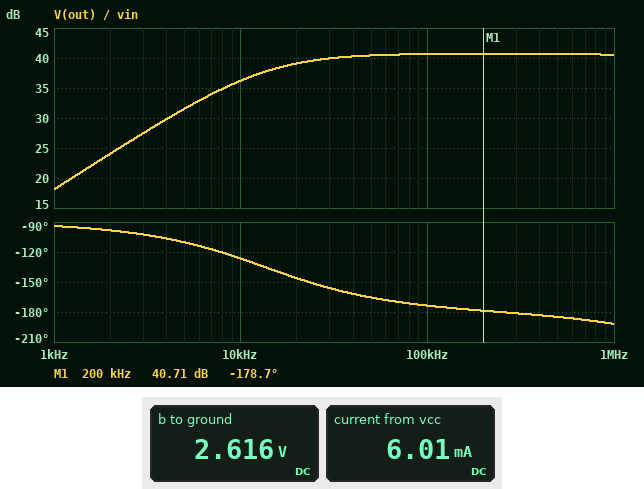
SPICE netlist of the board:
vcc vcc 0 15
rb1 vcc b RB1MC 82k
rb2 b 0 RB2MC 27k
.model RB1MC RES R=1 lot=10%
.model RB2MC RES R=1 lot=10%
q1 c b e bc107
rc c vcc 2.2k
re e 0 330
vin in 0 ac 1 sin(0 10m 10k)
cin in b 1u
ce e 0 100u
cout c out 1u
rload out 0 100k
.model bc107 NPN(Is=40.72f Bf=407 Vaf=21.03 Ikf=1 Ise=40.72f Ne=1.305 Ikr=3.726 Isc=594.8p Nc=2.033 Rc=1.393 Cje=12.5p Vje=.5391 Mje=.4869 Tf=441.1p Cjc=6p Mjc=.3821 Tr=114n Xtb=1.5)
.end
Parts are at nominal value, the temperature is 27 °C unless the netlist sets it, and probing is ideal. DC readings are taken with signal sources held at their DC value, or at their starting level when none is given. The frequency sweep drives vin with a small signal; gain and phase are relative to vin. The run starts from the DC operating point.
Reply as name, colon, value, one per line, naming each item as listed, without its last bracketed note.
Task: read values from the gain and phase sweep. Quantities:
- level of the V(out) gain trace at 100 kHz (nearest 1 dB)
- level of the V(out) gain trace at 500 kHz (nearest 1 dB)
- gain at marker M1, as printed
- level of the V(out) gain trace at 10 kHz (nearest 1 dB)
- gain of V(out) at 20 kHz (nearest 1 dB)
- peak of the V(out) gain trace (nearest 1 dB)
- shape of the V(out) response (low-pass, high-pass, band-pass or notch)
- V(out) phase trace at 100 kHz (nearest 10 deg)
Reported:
level of the V(out) gain trace at 100 kHz: 41 dB
level of the V(out) gain trace at 500 kHz: 41 dB
gain at marker M1, as printed: 40.71 dB
level of the V(out) gain trace at 10 kHz: 36 dB
gain of V(out) at 20 kHz: 39 dB
peak of the V(out) gain trace: 41 dB
shape of the V(out) response: high-pass
V(out) phase trace at 100 kHz: -170 deg
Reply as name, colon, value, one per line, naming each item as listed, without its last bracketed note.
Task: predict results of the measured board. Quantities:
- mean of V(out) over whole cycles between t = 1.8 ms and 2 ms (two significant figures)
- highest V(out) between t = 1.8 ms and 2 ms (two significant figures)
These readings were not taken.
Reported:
mean of V(out) over whole cycles between t = 1.8 ms and 2 ms: 2.0 V
highest V(out) between t = 1.8 ms and 2 ms: 4.5 V
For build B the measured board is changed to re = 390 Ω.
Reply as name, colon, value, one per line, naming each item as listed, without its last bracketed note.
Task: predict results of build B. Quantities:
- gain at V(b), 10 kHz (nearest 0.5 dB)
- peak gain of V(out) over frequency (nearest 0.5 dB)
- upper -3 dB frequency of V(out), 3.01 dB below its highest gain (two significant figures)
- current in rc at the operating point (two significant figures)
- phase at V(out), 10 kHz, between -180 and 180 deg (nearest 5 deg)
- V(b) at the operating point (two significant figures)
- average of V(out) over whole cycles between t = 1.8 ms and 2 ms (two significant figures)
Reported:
gain at V(b), 10 kHz: -2.5 dB
peak gain of V(out) over frequency: 45.0 dB
upper -3 dB frequency of V(out), 3.01 dB below its highest gain: 6.4 MHz
current in rc at the operating point: 5.7 mA
phase at V(out), 10 kHz, between -180 and 180 deg: -140 deg
V(b) at the operating point: 2.9 V
average of V(out) over whole cycles between t = 1.8 ms and 2 ms: 2.1 V
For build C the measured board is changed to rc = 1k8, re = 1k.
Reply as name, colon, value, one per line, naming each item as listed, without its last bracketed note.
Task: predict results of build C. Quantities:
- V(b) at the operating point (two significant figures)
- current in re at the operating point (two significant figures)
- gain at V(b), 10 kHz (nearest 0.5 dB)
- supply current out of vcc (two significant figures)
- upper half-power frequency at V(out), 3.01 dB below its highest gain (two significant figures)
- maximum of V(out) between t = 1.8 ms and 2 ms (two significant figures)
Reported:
V(b) at the operating point: 3.5 V
current in re at the operating point: 2.8 mA
gain at V(b), 10 kHz: 0 dB
supply current out of vcc: 3.0 mA
upper half-power frequency at V(out), 3.01 dB below its highest gain: 42 MHz
maximum of V(out) between t = 1.8 ms and 2 ms: 1.5 V
